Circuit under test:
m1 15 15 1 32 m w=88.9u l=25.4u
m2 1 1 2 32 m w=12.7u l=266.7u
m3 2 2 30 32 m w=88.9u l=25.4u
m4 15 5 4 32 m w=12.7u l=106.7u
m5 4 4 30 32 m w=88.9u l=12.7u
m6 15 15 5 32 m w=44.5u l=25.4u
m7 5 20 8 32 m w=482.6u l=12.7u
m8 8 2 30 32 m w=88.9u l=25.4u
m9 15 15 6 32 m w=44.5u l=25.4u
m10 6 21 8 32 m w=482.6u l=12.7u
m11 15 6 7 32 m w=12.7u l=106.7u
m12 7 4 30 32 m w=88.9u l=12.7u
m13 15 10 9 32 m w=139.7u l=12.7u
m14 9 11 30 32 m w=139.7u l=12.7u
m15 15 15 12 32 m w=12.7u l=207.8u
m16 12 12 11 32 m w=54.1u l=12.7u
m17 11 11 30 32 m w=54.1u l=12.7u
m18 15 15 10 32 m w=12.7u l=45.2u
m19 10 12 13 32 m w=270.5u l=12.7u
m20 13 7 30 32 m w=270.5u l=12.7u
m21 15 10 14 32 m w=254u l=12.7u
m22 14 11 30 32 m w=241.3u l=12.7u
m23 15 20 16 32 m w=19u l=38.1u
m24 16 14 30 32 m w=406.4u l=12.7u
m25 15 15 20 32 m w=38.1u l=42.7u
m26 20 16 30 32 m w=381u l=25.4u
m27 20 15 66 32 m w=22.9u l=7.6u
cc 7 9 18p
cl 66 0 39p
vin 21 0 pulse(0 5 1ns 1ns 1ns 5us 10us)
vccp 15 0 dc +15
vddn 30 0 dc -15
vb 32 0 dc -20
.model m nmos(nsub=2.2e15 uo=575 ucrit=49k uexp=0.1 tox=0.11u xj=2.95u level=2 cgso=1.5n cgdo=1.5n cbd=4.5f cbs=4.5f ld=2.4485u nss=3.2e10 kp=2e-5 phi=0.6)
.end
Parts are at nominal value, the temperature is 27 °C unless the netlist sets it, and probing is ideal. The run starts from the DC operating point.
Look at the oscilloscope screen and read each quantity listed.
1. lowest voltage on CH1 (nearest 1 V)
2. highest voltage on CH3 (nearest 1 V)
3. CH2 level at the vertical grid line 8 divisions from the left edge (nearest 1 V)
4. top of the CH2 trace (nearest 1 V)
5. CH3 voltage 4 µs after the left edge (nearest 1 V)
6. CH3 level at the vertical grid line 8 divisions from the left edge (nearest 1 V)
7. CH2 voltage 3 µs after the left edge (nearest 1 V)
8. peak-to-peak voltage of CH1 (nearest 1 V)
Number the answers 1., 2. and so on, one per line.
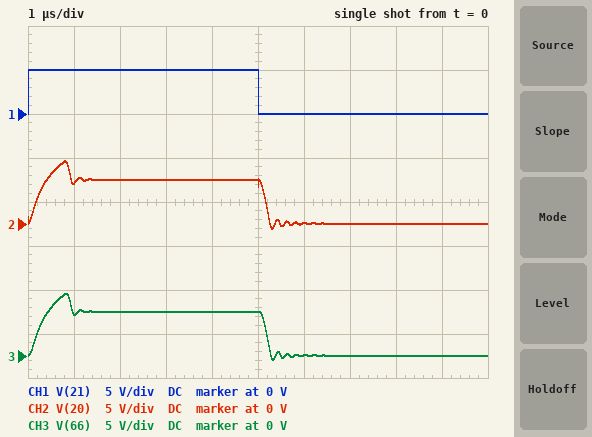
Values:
1. 0 V
2. 7 V
3. 0 V
4. 7 V
5. 5 V
6. 0 V
7. 5 V
8. 5 V
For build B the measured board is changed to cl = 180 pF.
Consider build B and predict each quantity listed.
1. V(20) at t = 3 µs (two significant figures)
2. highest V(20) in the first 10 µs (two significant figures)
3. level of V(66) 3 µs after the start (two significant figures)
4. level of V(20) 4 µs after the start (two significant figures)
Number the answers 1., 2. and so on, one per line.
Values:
1. 6.9 V
2. 7.0 V
3. 6.7 V
4. 5.0 V
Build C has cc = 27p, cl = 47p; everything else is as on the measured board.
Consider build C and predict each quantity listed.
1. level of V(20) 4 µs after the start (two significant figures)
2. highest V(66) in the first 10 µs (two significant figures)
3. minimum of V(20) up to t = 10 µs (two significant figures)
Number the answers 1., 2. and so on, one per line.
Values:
1. 5.0 V
2. 6.9 V
3. -320 mV
